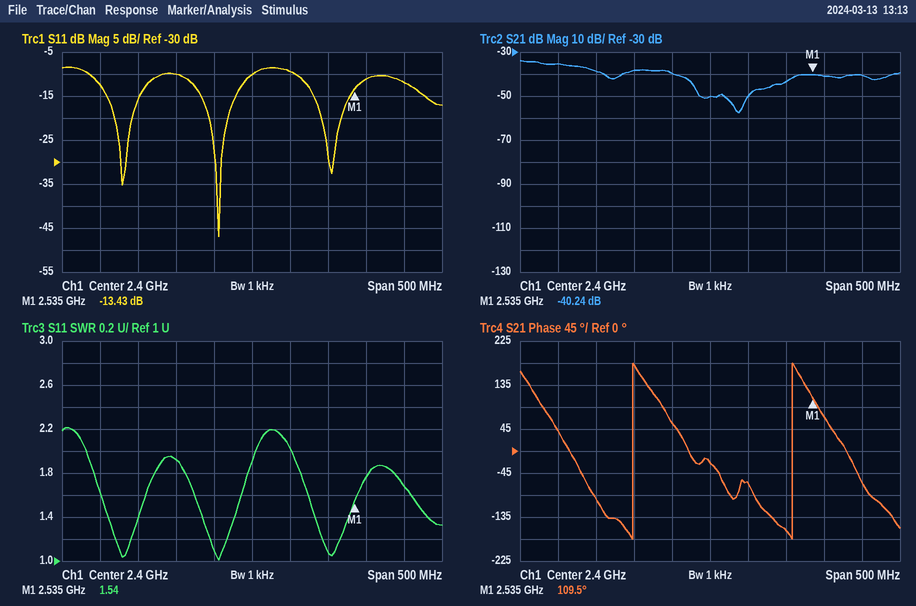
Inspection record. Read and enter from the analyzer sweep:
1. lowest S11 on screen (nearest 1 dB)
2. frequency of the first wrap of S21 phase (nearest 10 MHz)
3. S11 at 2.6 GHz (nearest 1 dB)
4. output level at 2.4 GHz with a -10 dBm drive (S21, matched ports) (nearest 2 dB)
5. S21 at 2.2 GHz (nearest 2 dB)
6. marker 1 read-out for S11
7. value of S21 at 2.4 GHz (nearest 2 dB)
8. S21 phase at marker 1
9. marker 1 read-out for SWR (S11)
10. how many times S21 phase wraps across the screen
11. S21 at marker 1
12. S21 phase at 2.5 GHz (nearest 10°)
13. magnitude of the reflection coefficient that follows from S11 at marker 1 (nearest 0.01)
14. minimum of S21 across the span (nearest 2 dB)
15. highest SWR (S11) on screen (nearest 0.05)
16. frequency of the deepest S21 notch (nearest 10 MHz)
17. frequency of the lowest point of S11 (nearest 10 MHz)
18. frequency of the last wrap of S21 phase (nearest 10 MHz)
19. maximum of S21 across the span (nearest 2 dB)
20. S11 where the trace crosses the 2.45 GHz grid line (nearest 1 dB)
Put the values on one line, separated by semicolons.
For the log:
-47 dB; 2.30 GHz; -12 dB; -60 dBm; -36 dB; -13.43 dB; -50 dB; 109.5°; 1.54; 2; -40.24 dB; -160°; 0.21; -58 dB; 2.20; 2.44 GHz; 2.36 GHz; 2.51 GHz; -34 dB; -9 dB
